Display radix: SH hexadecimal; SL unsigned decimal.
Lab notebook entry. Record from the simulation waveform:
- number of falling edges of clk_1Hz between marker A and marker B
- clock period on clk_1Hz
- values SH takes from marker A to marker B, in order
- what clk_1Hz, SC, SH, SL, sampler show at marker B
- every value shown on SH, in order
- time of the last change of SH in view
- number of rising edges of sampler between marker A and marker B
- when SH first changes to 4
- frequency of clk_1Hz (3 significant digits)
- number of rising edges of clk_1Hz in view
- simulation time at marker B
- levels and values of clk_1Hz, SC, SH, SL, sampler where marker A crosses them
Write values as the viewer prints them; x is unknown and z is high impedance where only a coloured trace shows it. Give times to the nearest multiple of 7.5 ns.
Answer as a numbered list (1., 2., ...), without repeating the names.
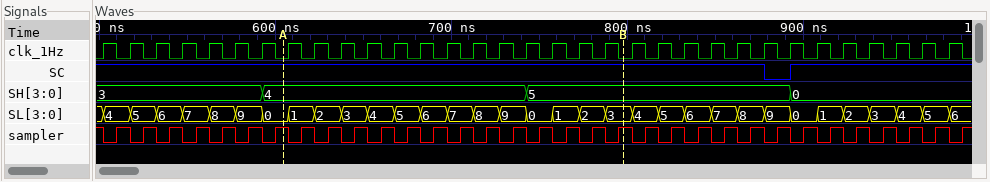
1. 13
2. 15 ns
3. 4, 5
4. clk_1Hz=0, SC=1, SH=5, SL=3, sampler=1
5. 3, 4, 5, 0
6. 892.5 ns
7. 13
8. 592.5 ns
9. 66.7 MHz
10. 33
11. 795 ns
12. clk_1Hz=0, SC=1, SH=4, SL=0, sampler=1
